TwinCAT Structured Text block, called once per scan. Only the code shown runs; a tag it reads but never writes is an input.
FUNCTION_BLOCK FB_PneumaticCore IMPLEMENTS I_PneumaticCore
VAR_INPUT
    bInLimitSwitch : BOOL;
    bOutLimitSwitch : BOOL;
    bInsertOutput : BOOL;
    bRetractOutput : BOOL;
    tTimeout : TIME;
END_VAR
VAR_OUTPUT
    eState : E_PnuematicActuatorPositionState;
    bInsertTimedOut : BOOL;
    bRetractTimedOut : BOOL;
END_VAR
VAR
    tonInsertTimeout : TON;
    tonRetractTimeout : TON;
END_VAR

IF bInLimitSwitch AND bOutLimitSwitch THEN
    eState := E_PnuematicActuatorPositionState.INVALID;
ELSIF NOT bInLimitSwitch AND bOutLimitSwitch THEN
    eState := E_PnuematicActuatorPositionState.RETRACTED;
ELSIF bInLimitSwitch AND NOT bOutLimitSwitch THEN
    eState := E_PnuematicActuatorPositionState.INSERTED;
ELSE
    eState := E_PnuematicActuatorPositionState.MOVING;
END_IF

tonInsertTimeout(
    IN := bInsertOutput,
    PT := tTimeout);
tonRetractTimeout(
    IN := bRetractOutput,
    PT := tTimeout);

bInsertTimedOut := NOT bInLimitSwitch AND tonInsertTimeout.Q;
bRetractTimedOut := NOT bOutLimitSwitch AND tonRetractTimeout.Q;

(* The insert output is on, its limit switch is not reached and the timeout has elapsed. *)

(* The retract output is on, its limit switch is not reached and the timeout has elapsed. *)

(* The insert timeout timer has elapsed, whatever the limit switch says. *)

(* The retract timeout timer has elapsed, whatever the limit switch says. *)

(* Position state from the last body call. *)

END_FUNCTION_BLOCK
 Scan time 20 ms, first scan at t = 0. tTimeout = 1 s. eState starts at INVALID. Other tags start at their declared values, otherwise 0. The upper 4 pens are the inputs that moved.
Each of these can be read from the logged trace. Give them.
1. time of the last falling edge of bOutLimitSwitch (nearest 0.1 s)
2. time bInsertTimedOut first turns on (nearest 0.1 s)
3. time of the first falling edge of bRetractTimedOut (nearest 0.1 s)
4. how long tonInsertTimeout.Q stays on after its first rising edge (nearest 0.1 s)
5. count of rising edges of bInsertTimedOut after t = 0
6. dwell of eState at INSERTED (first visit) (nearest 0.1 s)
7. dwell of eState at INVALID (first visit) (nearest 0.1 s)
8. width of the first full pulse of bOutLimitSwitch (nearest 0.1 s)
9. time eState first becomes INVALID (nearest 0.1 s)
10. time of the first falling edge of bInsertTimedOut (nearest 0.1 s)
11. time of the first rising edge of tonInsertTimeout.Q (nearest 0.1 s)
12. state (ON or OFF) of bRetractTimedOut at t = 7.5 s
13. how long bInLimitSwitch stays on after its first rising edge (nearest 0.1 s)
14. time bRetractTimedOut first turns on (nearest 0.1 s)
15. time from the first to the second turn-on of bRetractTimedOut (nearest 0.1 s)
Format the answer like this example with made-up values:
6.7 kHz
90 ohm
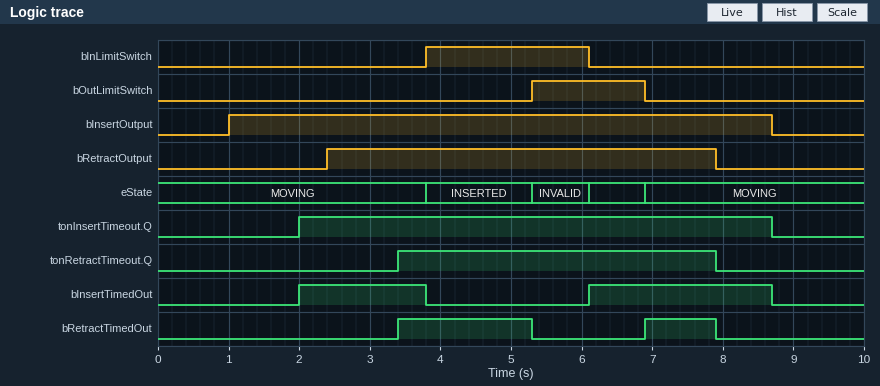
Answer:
6.9 s
2.0 s
5.3 s
6.7 s
2
1.5 s
0.8 s
1.6 s
5.3 s
3.8 s
2.0 s
ON
2.3 s
3.4 s
3.5 s
